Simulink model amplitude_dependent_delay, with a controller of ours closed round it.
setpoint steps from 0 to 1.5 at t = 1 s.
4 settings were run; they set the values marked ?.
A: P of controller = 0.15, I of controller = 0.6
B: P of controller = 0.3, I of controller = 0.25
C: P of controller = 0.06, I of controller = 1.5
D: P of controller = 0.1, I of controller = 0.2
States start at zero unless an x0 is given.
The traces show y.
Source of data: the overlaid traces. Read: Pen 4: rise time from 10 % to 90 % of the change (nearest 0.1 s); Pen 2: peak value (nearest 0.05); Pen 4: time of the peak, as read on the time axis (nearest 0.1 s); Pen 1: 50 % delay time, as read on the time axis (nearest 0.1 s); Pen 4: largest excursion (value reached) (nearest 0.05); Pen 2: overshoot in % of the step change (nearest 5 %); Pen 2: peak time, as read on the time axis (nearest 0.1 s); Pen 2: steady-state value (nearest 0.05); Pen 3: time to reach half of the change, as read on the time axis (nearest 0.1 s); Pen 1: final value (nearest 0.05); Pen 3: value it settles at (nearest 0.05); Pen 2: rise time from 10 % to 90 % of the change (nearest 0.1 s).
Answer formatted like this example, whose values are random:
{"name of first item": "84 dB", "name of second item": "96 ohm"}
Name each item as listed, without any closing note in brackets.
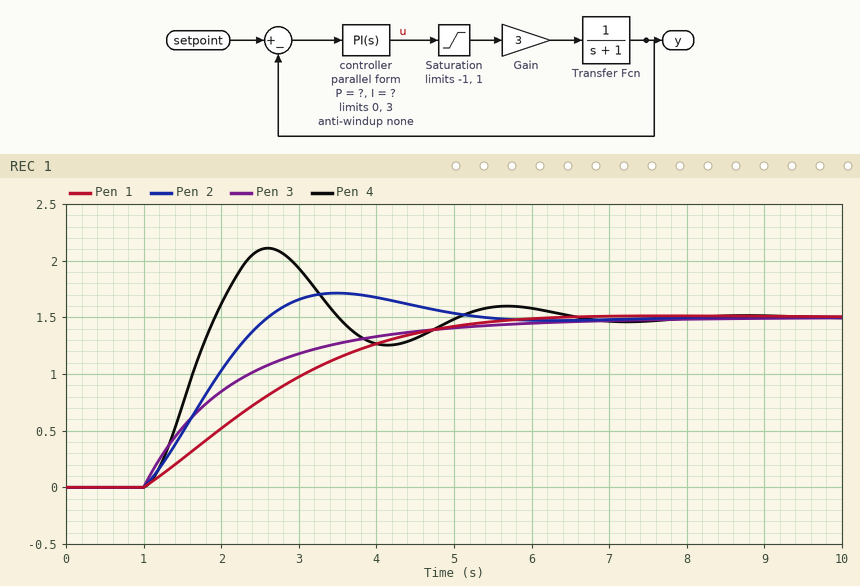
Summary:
{"Pen 4: rise time from 10 % to 90 % of the change": "0.6 s", "Pen 2: peak value": "1.70", "Pen 4: time of the peak, as read on the time axis": "2.6 s", "Pen 1: 50 % delay time, as read on the time axis": "2.5 s", "Pen 4: largest excursion (value reached)": "2.10", "Pen 2: overshoot in % of the step change": "15 %", "Pen 2: peak time, as read on the time axis": "3.5 s", "Pen 2: steady-state value": "1.50", "Pen 3: time to reach half of the change, as read on the time axis": "1.8 s", "Pen 1: final value": "1.50", "Pen 3: value it settles at": "1.50", "Pen 2: rise time from 10 % to 90 % of the change": "1.2 s"}
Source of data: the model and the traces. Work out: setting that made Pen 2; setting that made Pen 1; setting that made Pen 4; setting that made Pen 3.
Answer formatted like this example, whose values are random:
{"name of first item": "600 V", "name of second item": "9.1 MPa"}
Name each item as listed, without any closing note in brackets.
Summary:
{"setting that made Pen 2": "A", "setting that made Pen 1": "D", "setting that made Pen 4": "C", "setting that made Pen 3": "B"}
